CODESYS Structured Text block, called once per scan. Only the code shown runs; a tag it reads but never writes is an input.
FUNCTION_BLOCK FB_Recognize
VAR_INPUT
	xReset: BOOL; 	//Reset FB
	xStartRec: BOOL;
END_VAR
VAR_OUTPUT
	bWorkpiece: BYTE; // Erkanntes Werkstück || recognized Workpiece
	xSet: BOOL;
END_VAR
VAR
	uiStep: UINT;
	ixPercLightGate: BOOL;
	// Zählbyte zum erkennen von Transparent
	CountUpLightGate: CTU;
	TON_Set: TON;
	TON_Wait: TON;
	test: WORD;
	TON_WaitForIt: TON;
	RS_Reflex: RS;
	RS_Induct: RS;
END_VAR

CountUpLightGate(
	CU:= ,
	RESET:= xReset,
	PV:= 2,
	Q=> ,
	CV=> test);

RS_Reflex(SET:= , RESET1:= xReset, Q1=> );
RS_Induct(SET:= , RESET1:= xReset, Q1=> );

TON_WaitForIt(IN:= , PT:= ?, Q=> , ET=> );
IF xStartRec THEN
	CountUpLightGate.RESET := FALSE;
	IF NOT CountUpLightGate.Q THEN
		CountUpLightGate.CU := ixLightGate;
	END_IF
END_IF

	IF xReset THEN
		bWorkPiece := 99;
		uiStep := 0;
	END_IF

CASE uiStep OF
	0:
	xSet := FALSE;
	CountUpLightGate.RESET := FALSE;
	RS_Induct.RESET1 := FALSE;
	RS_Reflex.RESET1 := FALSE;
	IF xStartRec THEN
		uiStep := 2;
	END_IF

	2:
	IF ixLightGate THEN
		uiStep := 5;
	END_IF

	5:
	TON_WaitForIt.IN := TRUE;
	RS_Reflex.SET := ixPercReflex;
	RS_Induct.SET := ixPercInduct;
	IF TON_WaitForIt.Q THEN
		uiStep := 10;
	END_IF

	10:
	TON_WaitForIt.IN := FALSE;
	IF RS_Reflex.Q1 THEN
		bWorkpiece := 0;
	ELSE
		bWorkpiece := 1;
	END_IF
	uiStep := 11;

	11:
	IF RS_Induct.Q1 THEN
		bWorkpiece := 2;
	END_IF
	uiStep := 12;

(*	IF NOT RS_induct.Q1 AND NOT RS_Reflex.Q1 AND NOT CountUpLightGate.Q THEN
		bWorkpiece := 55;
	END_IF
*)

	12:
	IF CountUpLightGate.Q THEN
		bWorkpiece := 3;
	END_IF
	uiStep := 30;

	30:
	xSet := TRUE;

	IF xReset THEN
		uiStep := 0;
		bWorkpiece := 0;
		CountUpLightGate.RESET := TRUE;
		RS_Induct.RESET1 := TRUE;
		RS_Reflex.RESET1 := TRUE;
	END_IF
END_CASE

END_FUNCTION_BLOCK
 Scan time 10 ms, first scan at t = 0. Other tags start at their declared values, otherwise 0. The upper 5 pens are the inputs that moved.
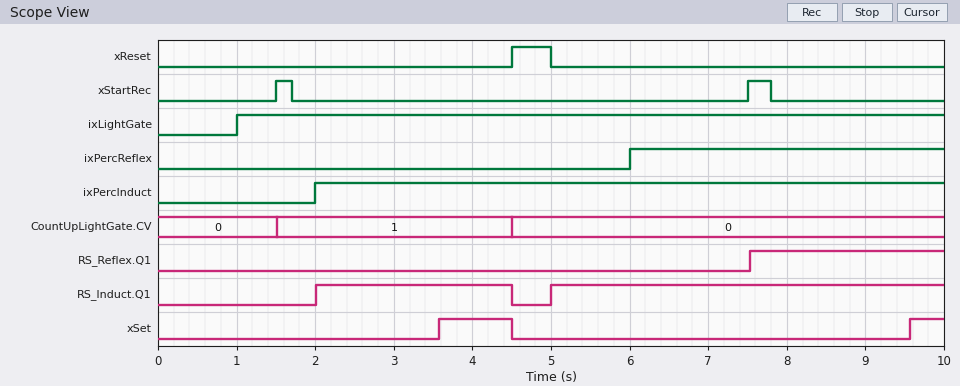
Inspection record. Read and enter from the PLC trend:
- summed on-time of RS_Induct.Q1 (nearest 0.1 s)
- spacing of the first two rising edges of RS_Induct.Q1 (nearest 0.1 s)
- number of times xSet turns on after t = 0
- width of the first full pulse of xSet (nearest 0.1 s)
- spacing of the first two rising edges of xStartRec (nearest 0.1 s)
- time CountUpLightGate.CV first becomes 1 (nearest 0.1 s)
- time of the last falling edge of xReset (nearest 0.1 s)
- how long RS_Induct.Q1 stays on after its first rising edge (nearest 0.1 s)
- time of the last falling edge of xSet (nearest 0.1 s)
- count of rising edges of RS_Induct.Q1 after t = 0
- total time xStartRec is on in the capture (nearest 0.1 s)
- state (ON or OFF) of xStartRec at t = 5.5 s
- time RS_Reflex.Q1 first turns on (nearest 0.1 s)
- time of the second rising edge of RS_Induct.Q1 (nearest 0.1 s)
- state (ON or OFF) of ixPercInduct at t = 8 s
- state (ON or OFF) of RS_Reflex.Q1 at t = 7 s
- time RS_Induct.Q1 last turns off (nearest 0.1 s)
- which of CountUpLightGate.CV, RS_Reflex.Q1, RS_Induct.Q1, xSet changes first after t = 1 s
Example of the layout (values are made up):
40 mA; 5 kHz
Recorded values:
7.5 s; 3.0 s; 2; 0.9 s; 6.0 s; 1.5 s; 5.0 s; 2.5 s; 4.5 s; 2; 0.5 s; OFF; 7.5 s; 5.0 s; ON; OFF; 4.5 s; CountUpLightGate.CV
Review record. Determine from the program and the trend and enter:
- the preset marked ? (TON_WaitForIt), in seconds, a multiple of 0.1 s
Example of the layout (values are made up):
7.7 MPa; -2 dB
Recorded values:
2.0 s
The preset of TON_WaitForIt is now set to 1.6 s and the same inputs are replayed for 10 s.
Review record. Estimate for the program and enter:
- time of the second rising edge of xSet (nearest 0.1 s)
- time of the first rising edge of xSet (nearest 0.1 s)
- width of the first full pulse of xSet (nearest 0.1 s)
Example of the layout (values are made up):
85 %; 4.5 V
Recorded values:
9.2 s; 3.2 s; 1.3 s
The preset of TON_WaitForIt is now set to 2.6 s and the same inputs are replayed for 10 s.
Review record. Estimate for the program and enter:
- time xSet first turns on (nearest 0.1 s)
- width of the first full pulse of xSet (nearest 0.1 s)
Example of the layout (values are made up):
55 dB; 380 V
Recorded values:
4.2 s; 0.3 s
